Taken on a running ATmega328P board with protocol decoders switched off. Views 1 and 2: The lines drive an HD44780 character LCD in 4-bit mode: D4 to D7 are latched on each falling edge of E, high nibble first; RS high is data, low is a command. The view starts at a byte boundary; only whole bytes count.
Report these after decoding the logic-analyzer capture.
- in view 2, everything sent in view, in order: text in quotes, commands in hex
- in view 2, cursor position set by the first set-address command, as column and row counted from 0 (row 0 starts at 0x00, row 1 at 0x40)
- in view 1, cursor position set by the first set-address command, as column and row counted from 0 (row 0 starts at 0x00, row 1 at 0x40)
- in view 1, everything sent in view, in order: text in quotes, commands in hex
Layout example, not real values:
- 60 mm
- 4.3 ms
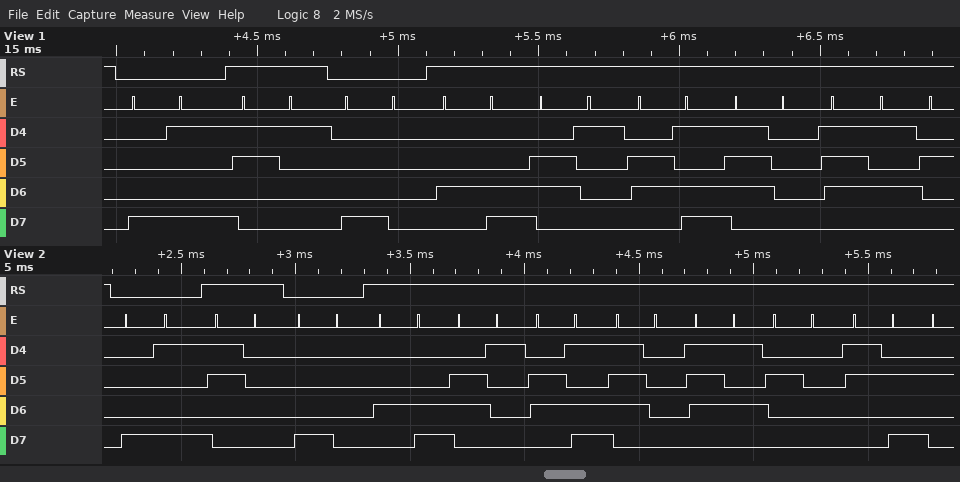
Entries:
- 0x89 "0" 0x80 "Lampu :"
- column 9, row 0
- column 9, row 0
- 0x89 "1" 0x80 "Lampu"
